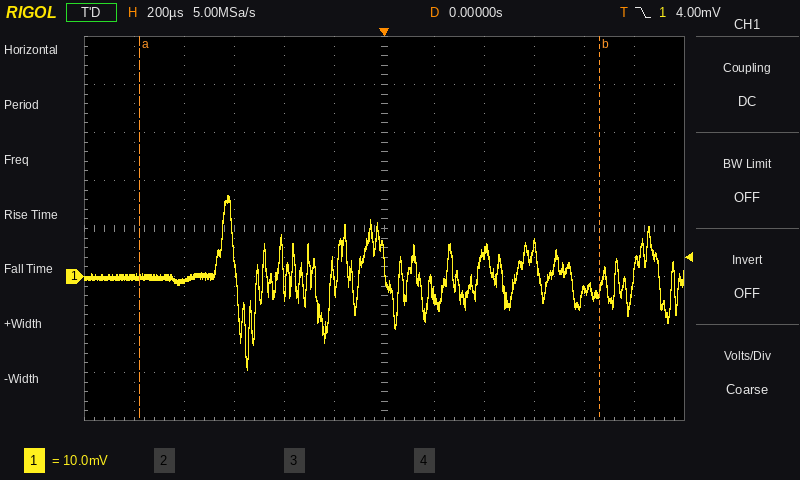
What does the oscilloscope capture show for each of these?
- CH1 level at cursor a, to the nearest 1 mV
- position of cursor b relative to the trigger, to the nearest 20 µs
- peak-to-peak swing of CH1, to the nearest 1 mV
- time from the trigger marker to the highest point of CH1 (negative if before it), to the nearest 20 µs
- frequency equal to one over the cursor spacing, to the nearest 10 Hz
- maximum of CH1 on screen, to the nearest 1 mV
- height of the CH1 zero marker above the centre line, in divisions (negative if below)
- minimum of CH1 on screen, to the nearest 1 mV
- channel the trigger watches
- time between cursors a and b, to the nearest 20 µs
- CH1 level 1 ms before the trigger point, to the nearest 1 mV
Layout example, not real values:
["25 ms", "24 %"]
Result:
["0 mV", "+860 µs", "36 mV", "-620 µs", "540 Hz", "17 mV", "-1.0 div", "-19 mV", "CH1", "1.84 ms", "0 mV"]
